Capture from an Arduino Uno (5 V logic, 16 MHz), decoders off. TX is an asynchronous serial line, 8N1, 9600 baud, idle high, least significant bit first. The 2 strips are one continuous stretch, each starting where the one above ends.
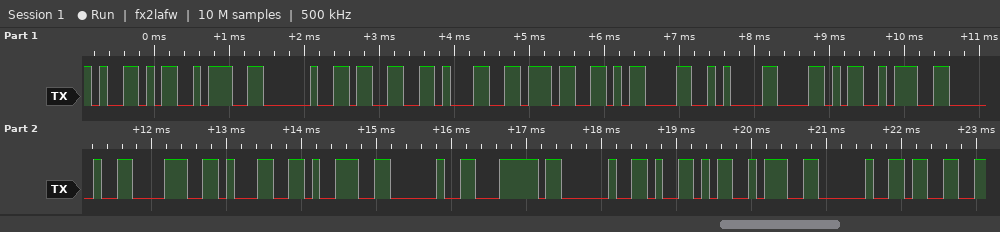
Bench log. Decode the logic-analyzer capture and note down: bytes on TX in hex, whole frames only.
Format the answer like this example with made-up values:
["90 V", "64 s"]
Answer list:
["0x59 0x3A 0x20 0x33 0x31 0x37 0x0D 0x0A 0x58 0x3A 0x20 0x38 0x31 0x39 0x20 0x7C 0x20 0x59 0x3A 0x20 0x33"]
